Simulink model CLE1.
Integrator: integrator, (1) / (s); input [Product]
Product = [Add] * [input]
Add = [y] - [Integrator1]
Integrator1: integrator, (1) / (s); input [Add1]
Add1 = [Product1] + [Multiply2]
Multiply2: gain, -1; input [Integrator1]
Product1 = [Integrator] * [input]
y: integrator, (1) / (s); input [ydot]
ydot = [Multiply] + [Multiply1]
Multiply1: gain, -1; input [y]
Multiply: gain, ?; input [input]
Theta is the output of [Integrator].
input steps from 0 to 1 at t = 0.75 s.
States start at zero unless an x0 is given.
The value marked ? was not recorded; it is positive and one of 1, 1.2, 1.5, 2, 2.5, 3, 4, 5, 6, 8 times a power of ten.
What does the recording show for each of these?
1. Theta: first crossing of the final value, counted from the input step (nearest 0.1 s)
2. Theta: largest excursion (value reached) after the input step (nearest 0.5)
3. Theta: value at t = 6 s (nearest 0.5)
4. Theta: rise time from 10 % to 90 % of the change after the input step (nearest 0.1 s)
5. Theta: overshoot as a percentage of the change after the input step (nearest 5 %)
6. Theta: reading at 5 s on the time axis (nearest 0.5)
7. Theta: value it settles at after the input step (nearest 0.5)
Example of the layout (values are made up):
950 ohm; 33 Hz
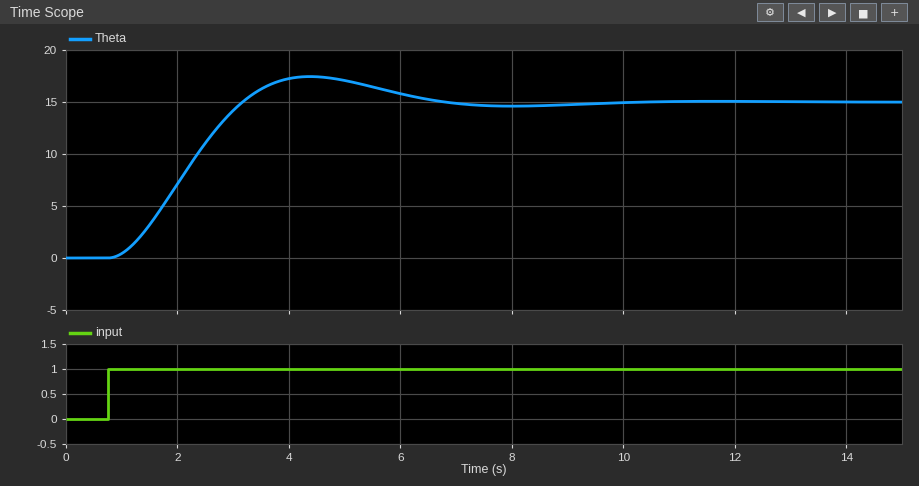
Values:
2.4 s; 17.5; 16.0; 1.6 s; 15 %; 17.0; 15.0
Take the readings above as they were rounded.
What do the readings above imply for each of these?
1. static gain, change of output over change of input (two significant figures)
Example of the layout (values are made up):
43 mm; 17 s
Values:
15
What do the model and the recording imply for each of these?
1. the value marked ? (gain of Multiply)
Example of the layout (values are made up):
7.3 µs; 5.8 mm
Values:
15
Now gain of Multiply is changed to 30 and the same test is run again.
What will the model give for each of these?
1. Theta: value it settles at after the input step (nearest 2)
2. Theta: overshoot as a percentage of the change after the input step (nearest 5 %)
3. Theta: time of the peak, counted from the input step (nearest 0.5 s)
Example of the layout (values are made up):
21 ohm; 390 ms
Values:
30; 15 %; 3.5 s
